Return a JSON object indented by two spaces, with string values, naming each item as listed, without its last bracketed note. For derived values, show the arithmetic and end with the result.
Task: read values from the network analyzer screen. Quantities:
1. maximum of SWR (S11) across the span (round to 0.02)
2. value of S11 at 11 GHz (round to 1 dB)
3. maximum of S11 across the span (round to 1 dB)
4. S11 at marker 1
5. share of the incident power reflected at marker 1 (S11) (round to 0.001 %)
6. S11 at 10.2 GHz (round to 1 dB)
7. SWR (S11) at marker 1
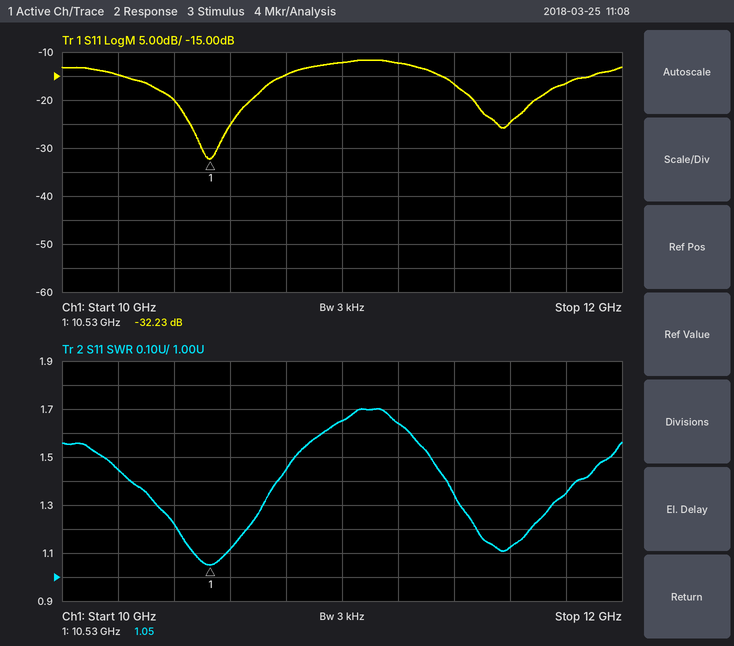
{
  "maximum of SWR (S11) across the span": "1.70",
  "value of S11 at 11 GHz": "-12 dB",
  "maximum of S11 across the span": "-12 dB",
  "S11 at marker 1": "-32.23 dB",
  "share of the incident power reflected at marker 1 (S11)": "10^(-32.23/10) ≈ 0.060 %",
  "S11 at 10.2 GHz": "-15 dB",
  "SWR (S11) at marker 1": "1.05"
}
